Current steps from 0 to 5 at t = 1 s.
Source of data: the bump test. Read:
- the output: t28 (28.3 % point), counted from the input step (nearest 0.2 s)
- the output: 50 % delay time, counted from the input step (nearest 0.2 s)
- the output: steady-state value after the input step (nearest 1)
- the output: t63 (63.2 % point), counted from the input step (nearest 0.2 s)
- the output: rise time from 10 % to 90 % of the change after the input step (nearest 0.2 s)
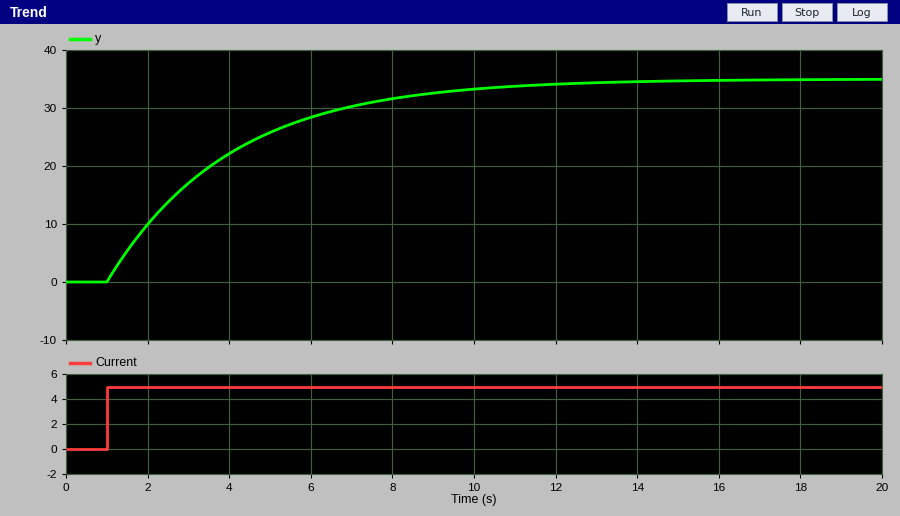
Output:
1.0 s
2.0 s
35
3.0 s
6.6 s
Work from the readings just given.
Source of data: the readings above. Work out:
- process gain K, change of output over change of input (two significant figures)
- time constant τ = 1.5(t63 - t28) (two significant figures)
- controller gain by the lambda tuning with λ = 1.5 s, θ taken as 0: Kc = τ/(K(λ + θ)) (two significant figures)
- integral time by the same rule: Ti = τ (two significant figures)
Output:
7.0
3.0 s
0.29
3.0 s
